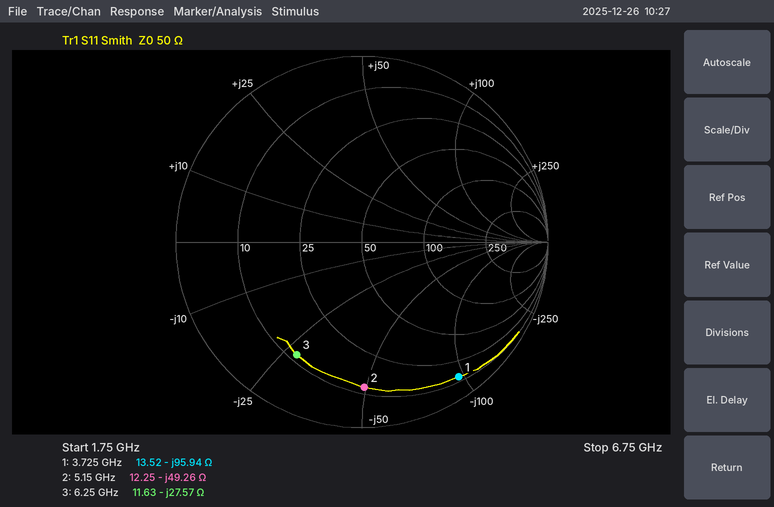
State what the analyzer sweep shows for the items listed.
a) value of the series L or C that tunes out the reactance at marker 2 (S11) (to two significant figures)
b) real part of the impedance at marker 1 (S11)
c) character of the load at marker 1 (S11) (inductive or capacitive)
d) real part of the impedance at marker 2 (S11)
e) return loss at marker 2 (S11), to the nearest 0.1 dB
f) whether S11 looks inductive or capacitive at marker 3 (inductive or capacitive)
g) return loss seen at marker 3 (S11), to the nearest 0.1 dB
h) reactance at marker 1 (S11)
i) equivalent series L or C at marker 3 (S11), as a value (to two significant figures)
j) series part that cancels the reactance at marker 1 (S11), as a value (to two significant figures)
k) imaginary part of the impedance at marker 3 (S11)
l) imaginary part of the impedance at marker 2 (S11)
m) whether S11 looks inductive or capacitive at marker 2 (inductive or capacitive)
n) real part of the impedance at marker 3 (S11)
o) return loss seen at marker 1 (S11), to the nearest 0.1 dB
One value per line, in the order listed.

1.5 nH
13.52 Ω
capacitive
12.25 Ω
2.1 dB
capacitive
3.1 dB
-95.94 Ω
920 fF
4.1 nH
-27.57 Ω
-49.26 Ω
capacitive
11.63 Ω
1.0 dB
